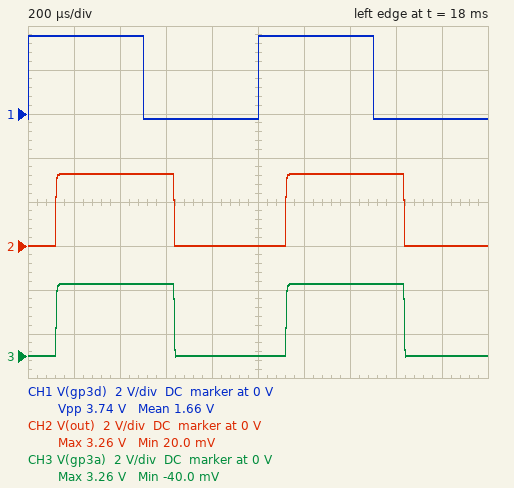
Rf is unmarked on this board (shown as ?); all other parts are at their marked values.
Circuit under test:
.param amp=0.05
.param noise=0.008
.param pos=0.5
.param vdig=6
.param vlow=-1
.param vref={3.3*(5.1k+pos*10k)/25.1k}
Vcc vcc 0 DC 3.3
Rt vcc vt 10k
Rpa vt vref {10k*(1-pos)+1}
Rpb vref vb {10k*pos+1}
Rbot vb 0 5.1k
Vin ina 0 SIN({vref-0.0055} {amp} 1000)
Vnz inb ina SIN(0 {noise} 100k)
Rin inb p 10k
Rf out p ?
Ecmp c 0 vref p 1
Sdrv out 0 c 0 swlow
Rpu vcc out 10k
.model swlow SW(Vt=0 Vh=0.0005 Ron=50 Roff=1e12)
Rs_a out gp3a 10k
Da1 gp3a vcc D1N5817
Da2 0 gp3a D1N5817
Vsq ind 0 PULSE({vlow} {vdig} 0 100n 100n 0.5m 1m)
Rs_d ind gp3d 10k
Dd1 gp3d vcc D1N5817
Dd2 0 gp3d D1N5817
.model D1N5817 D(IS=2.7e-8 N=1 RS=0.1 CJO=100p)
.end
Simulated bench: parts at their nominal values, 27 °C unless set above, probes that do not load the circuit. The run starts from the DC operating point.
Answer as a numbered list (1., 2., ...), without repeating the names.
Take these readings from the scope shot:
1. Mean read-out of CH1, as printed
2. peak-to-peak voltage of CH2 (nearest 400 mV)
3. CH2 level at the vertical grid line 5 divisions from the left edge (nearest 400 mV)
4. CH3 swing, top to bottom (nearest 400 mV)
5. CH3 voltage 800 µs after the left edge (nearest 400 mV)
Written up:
1. 1.66 V
2. 3.2 V
3. 0 V
4. 3.2 V
5. 0 V
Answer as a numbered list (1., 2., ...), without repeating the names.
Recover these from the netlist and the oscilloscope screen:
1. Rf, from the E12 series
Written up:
1. 390 kΩ
